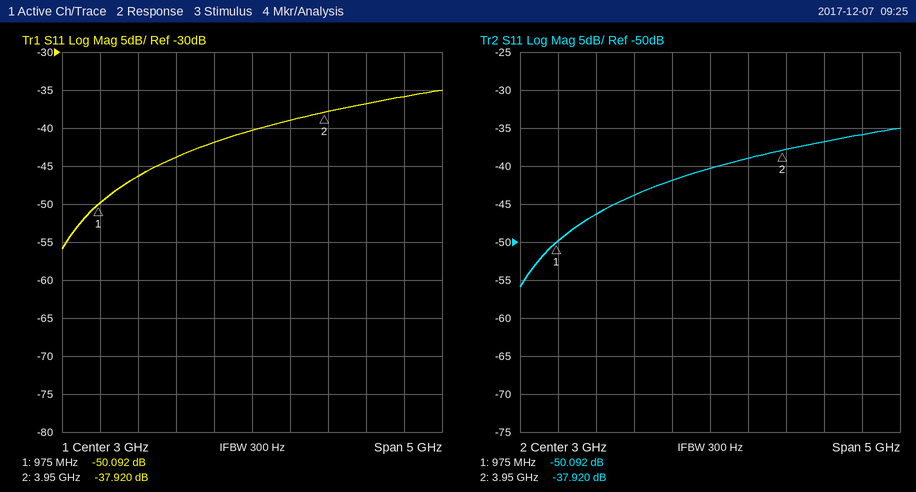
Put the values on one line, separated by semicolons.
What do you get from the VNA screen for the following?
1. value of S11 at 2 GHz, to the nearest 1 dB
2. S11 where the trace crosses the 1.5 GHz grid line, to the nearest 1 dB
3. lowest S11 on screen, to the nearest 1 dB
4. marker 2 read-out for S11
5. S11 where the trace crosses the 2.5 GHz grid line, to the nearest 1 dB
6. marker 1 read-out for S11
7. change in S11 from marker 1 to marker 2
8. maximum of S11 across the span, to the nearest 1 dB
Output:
-44 dB; -46 dB; -56 dB; -37.920 dB; -42 dB; -50.092 dB; 12.172 dB; -35 dB
